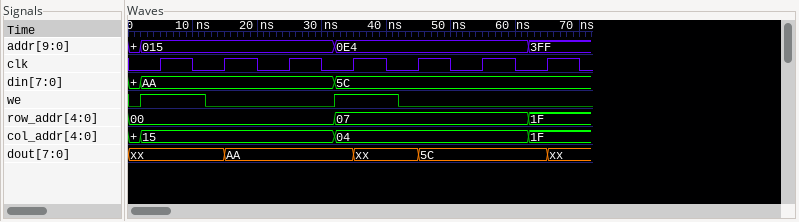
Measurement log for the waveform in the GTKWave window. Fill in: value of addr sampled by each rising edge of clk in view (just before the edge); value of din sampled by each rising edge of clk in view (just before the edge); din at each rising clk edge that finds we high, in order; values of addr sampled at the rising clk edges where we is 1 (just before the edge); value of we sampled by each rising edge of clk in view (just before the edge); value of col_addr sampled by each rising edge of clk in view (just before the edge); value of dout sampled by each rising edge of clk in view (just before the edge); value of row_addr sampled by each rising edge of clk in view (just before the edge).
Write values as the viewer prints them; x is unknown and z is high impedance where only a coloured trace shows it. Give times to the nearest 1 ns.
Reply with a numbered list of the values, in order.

1. 015, 015, 015, 0E4, 0E4, 0E4, 3FF
2. AA, AA, AA, 5C, 5C, 5C, 5C
3. AA, 5C
4. 015, 0E4
5. 1 0 0 1 0 0 0
6. 15, 15, 15, 04, 04, 04, 1F
7. xx, xx, AA, AA, xx, 5C, 5C
8. 00, 00, 00, 07, 07, 07, 1F
